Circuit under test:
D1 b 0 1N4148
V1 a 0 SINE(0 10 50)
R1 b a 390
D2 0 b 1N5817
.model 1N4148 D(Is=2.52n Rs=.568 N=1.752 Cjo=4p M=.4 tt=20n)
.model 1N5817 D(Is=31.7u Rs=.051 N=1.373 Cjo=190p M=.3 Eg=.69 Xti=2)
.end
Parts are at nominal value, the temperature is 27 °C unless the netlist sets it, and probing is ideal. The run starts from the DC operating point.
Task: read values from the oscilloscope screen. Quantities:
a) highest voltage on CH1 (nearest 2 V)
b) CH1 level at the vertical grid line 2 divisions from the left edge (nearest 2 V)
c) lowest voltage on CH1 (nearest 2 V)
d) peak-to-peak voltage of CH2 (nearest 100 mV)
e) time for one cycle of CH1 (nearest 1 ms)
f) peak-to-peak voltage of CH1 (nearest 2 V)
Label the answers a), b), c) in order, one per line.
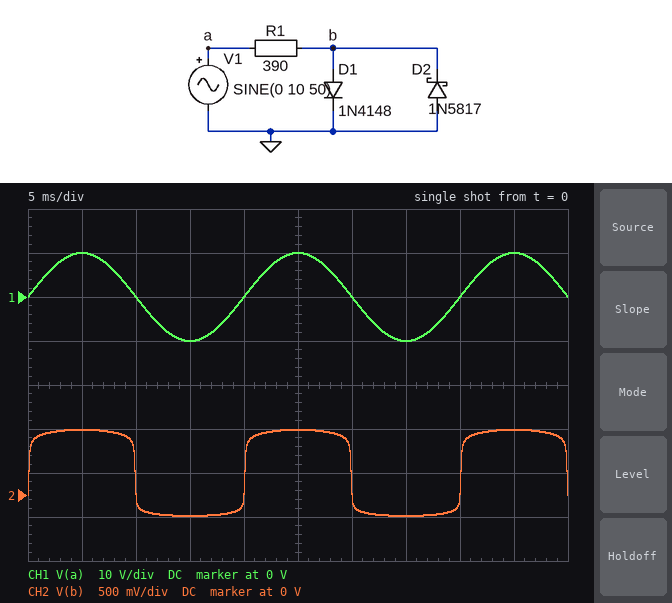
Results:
a) 10 V
b) 0 V
c) -10 V
d) 1.0 V
e) 20 ms
f) 20 V
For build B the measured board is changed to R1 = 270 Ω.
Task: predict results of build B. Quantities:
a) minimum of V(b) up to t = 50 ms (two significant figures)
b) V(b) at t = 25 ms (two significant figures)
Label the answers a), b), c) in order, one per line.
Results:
a) -250 mV
b) 760 mV
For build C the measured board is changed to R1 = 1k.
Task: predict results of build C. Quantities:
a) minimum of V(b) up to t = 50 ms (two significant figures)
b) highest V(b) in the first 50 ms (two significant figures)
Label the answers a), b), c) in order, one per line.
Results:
a) -200 mV
b) 690 mV
